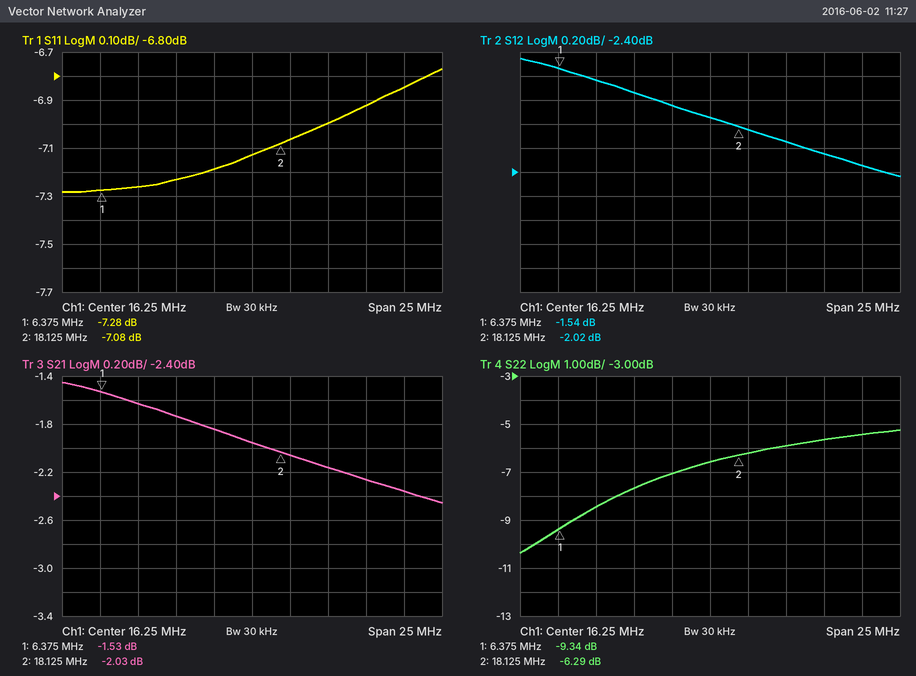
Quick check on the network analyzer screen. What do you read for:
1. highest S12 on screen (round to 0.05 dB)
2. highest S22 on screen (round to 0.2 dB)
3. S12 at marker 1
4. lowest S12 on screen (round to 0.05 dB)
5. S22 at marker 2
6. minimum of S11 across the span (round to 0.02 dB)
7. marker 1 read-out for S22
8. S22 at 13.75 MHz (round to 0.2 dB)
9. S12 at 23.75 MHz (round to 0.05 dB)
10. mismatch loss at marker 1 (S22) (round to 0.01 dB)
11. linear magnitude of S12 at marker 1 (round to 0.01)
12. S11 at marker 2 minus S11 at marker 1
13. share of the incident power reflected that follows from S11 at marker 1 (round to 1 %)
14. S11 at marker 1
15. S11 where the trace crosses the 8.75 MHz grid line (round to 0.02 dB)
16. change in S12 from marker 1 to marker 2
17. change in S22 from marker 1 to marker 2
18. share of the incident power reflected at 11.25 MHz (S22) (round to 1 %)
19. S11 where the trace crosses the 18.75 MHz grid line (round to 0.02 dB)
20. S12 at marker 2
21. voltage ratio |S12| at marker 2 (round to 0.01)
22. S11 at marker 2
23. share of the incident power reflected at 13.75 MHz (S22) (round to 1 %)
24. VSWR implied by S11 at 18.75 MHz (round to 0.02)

-1.45 dB
-5.2 dB
-1.54 dB
-2.45 dB
-6.29 dB
-7.28 dB
-9.34 dB
-7.0 dB
-2.25 dB
0.54 dB
0.84
0.20 dB
19 %
-7.28 dB
-7.26 dB
-0.48 dB
3.05 dB
17 %
-7.06 dB
-2.02 dB
0.79
-7.08 dB
20 %
2.60
